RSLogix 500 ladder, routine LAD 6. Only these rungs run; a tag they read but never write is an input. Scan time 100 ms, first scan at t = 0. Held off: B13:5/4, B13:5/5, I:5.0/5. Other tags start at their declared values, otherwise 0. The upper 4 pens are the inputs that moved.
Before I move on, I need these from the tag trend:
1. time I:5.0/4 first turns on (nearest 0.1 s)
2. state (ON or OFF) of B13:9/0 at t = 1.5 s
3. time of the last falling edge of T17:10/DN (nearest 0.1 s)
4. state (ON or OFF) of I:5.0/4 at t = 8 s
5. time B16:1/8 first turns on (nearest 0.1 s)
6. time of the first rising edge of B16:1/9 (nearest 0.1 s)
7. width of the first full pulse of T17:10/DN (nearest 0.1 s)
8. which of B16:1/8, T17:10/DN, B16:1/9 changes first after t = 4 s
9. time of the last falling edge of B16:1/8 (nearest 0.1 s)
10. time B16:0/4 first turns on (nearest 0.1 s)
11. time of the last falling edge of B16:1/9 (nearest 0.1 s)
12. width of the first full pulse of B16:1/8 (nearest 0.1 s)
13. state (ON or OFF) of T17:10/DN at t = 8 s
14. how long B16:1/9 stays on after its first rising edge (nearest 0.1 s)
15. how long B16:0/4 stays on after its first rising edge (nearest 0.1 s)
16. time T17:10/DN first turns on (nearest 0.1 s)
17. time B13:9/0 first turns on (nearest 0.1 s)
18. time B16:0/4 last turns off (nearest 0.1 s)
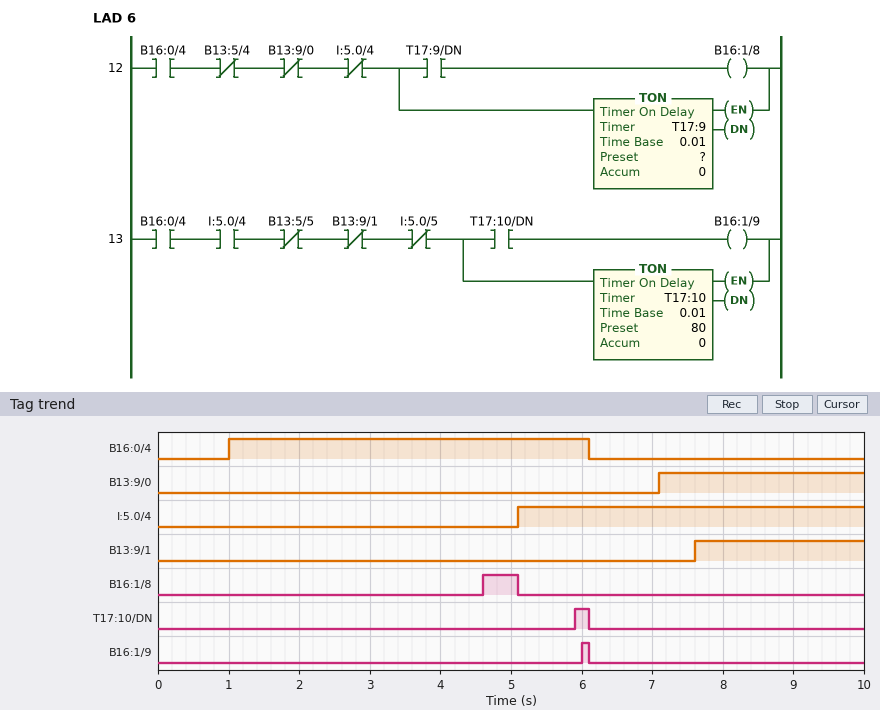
5.1 s
OFF
6.1 s
ON
4.6 s
6.0 s
0.2 s
B16:1/8
5.1 s
1.0 s
6.1 s
0.5 s
OFF
0.1 s
5.1 s
5.9 s
7.1 s
6.1 s
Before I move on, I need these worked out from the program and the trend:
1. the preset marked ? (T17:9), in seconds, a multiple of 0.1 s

3.5 s
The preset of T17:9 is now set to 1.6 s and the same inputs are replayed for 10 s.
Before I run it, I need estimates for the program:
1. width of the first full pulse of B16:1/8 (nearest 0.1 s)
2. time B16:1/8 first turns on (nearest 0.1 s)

2.4 s
2.7 s
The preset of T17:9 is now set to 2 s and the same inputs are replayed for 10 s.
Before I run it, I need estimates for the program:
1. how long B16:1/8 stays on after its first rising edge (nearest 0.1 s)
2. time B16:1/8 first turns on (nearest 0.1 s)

2.0 s
3.1 s
